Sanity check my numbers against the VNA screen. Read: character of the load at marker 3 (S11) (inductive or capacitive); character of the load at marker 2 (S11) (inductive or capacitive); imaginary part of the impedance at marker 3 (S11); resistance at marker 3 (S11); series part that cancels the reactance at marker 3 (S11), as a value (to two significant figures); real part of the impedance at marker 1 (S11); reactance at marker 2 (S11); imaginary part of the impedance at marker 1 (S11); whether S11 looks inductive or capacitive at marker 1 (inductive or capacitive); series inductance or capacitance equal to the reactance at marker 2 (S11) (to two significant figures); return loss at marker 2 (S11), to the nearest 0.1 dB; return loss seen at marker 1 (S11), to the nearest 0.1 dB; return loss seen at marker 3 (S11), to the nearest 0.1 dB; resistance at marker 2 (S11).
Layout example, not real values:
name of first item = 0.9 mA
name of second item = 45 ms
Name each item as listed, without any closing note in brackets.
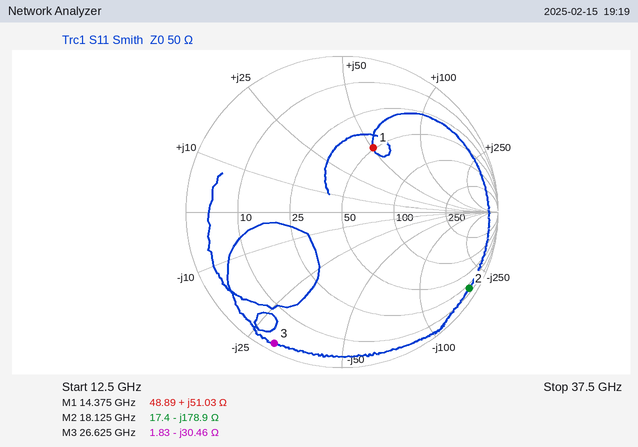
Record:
character of the load at marker 3 (S11) = capacitive
character of the load at marker 2 (S11) = capacitive
imaginary part of the impedance at marker 3 = -30.46 Ω
resistance at marker 3 = 1.83 Ω
series part that cancels the reactance at marker 3 (S11), as a value = 180 pH
real part of the impedance at marker 1 = 48.89 Ω
reactance at marker 2 = -178.9 Ω
imaginary part of the impedance at marker 1 = +51.03 Ω
whether S11 looks inductive or capacitive at marker 1 = inductive
series inductance or capacitance equal to the reactance at marker 2 (S11) = 49 fF
return loss at marker 2 (S11), to the nearest 0.1 dB = 0.4 dB
return loss seen at marker 1 (S11), to the nearest 0.1 dB = 6.8 dB
return loss seen at marker 3 (S11), to the nearest 0.1 dB = 0.5 dB
resistance at marker 2 = 17.4 Ω
